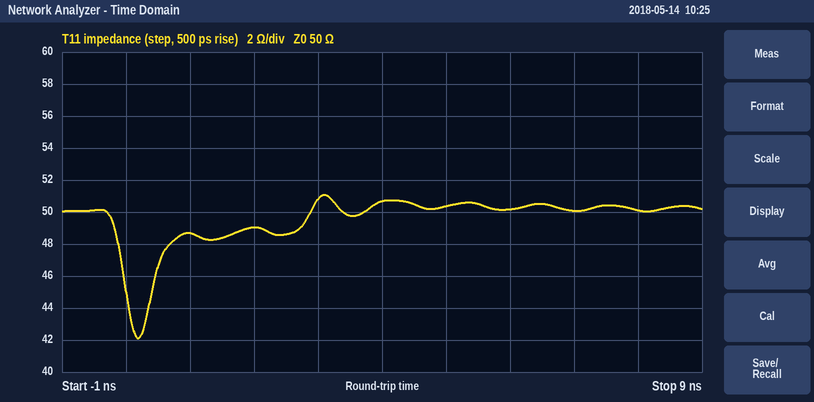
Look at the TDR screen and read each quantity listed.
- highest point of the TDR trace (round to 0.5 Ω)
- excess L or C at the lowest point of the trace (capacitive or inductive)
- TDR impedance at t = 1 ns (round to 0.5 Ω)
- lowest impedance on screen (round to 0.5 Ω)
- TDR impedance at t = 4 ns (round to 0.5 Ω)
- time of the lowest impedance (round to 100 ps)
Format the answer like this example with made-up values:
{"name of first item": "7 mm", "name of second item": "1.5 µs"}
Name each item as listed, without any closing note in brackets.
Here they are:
{"highest point of the TDR trace": "51.0 Ω", "excess L or C at the lowest point of the trace": "capacitive", "TDR impedance at t = 1 ns": "48.5 Ω", "lowest impedance on screen": "42.0 Ω", "TDR impedance at t = 4 ns": "50.5 Ω", "time of the lowest impedance": "200 ps"}
